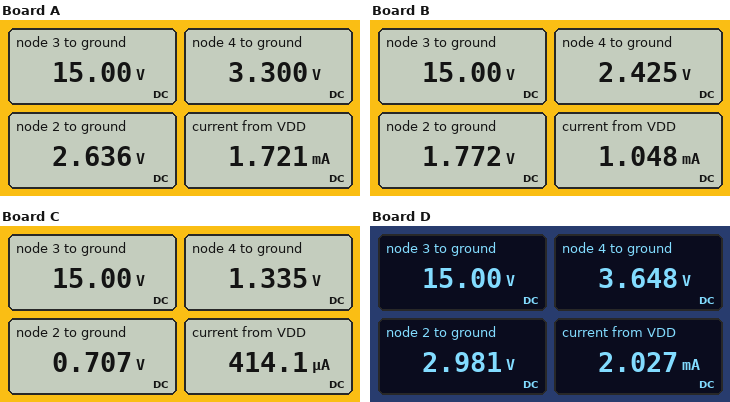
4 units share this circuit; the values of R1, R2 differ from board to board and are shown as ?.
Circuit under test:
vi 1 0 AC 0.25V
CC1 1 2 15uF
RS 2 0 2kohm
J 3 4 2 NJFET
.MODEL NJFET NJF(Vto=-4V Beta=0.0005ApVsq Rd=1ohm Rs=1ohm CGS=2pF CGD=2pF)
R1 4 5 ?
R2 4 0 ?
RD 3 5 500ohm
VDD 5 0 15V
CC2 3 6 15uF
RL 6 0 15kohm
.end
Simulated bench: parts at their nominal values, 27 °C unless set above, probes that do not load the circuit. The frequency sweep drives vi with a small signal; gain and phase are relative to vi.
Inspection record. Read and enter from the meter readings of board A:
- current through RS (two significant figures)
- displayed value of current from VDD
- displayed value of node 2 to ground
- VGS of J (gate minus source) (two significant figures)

1.3 mA
1.721 mA
2.636 V
660 mV
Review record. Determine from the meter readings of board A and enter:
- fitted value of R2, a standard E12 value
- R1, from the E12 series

8.2 kΩ
6.8 kΩ
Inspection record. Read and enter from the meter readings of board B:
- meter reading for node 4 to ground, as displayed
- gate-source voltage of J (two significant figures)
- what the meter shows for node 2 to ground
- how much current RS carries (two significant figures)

2.425 V
650 mV
1.772 V
890 µA
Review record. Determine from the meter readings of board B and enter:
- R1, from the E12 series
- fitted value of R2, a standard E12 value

12 kΩ
15 kΩ
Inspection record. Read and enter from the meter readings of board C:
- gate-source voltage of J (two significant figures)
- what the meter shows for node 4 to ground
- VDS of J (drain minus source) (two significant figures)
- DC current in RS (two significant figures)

630 mV
1.335 V
14 V
350 µA
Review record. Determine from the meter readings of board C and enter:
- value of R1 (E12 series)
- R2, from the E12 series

33 kΩ
22 kΩ
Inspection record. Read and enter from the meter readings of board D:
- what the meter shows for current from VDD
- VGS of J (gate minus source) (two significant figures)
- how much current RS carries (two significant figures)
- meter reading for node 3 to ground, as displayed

2.027 mA
670 mV
1.5 mA
15.00 V
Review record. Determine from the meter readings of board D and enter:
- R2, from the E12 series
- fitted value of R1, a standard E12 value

6.8 kΩ
5.6 kΩ
